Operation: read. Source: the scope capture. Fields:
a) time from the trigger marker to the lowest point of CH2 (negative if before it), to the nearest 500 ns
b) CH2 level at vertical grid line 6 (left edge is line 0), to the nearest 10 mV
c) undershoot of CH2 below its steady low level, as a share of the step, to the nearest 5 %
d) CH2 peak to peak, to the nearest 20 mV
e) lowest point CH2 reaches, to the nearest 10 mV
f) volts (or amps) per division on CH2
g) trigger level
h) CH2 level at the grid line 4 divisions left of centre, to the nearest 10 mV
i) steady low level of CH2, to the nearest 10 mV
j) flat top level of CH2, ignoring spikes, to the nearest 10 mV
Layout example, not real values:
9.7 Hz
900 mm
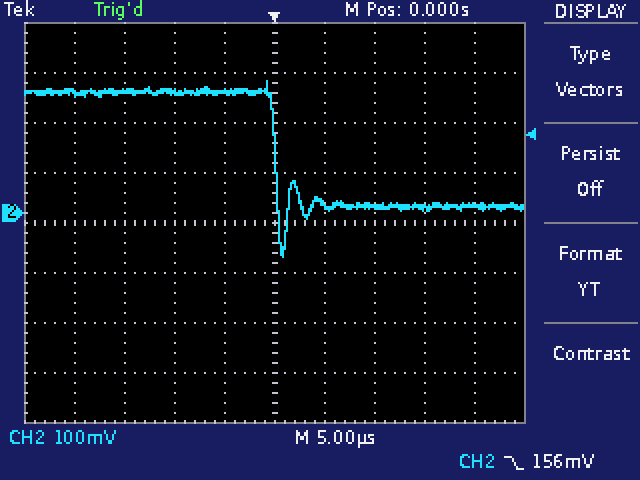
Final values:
+1.0 µs
20 mV
45 %
360 mV
-90 mV
100 mV
156 mV
240 mV
10 mV
240 mV
